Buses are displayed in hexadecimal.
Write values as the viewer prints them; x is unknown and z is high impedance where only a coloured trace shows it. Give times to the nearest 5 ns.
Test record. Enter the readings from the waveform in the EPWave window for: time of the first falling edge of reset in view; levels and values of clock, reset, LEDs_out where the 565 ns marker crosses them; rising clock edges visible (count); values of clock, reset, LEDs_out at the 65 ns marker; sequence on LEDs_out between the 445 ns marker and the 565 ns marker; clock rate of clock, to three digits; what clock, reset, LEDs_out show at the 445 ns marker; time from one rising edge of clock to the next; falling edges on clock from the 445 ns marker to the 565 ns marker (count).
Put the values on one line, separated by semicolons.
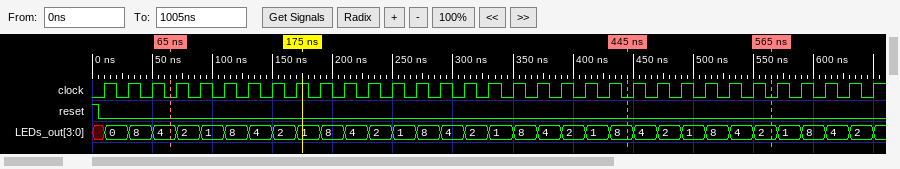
5 ns; clock=0, reset=0, LEDs_out=2; 33; clock=0, reset=0, LEDs_out=4; 8, 4, 2, 1, 8, 4, 2; 50.0 MHz; clock=0, reset=0, LEDs_out=8; 20 ns; 6
